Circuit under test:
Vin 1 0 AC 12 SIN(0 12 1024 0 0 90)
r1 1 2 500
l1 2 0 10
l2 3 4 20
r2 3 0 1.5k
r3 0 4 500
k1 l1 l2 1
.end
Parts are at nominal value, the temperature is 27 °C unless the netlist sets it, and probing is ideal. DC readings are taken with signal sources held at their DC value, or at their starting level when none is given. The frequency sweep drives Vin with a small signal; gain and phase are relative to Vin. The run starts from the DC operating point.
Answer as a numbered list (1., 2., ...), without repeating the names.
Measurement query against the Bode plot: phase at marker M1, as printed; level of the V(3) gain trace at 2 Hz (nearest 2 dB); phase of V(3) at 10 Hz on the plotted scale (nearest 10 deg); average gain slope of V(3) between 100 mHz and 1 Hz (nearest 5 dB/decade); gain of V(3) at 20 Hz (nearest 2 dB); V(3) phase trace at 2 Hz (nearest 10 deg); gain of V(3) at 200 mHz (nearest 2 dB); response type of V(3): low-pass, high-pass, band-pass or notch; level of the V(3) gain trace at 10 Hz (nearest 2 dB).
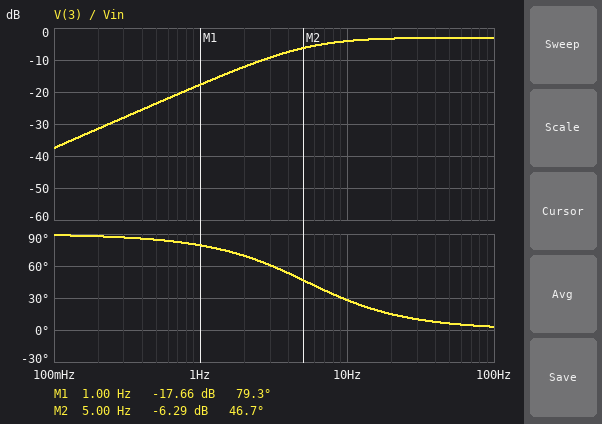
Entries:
1. 79.3 deg
2. -12 dB
3. 30 deg
4. 20 dB/decade
5. -4 dB
6. 70 deg
7. -32 dB
8. high-pass
9. -4 dB
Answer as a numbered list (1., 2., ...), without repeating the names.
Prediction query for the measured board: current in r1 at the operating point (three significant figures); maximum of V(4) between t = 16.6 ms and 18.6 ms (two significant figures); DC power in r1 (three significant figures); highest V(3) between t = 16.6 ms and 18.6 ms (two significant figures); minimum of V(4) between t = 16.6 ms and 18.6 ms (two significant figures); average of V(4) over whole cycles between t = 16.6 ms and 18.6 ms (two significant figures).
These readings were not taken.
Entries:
1. 24.0 mA
2. 4.4 V
3. 288 mW
4. 3.9 V
5. -1.3 V
6. 1.6 V
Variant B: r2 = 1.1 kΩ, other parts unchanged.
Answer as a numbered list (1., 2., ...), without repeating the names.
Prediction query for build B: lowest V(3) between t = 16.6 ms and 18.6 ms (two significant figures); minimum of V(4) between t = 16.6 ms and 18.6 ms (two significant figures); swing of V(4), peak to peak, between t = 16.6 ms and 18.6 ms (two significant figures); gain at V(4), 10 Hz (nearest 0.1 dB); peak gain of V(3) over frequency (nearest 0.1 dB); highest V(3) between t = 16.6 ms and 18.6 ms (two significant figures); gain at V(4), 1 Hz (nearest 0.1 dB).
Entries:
1. -11 V
2. -1.4 V
3. 6.6 V
4. -12.2 dB
5. -4.5 dB
6. 3.1 V
7. -25.3 dB
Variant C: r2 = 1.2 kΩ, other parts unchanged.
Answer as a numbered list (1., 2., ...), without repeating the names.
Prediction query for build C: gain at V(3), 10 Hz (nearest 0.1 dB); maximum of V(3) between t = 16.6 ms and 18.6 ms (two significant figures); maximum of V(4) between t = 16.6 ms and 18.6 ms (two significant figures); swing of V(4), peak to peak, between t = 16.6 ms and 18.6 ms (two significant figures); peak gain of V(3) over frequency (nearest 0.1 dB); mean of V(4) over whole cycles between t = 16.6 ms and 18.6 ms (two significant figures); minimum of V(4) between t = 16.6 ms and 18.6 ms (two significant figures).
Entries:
1. -5.0 dB
2. 3.3 V
3. 5.0 V
4. 6.4 V
5. -4.0 dB
6. 1.8 V
7. -1.4 V
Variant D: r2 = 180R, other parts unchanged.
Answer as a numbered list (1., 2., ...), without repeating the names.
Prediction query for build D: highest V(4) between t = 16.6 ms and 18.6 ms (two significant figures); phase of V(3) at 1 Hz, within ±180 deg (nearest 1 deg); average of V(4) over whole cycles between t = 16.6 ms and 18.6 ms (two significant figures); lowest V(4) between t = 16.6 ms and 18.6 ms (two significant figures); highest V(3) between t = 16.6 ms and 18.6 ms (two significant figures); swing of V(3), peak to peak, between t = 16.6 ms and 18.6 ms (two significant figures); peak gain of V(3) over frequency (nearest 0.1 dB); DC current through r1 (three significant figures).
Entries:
1. 8.6 V
2. 73 deg
3. 3.5 V
4. -1.6 V
5. 570 mV
6. 3.7 V
7. -16.4 dB
8. 24.0 mA
